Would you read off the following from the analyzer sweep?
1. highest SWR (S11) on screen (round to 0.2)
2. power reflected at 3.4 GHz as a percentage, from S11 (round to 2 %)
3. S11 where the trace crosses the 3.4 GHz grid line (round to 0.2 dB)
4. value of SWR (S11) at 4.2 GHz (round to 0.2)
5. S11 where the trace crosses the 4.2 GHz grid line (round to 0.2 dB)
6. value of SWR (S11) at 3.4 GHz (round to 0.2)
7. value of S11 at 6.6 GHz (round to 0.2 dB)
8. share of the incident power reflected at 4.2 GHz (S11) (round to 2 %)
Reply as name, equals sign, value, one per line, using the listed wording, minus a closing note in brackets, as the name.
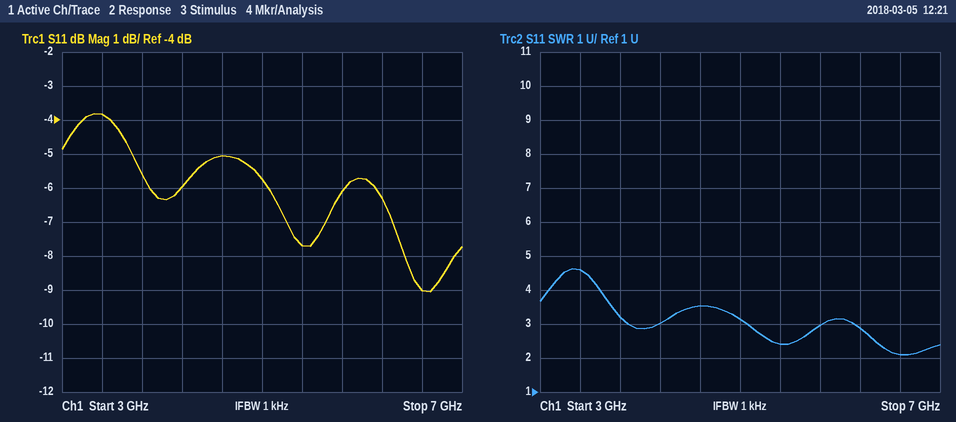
highest SWR (S11) on screen = 4.6
power reflected at 3.4 GHz as a percentage, from S11 = 42 %
S11 where the trace crosses the 3.4 GHz grid line = -3.8 dB
value of SWR (S11) at 4.2 GHz = 3.0
S11 where the trace crosses the 4.2 GHz grid line = -6.0 dB
value of SWR (S11) at 3.4 GHz = 4.6
value of S11 at 6.6 GHz = -9.0 dB
share of the incident power reflected at 4.2 GHz (S11) = 26 %
